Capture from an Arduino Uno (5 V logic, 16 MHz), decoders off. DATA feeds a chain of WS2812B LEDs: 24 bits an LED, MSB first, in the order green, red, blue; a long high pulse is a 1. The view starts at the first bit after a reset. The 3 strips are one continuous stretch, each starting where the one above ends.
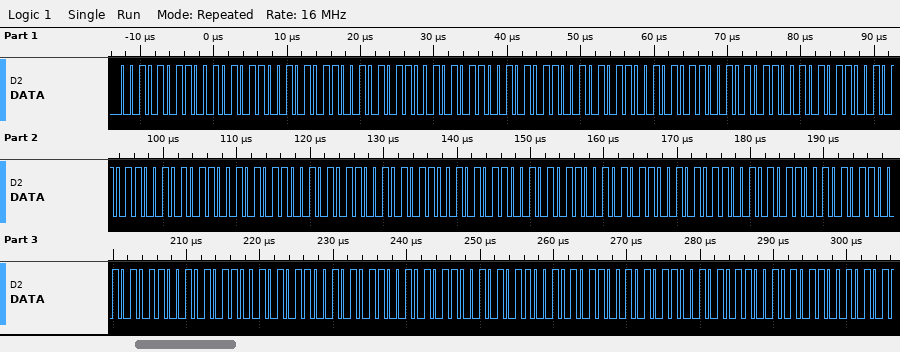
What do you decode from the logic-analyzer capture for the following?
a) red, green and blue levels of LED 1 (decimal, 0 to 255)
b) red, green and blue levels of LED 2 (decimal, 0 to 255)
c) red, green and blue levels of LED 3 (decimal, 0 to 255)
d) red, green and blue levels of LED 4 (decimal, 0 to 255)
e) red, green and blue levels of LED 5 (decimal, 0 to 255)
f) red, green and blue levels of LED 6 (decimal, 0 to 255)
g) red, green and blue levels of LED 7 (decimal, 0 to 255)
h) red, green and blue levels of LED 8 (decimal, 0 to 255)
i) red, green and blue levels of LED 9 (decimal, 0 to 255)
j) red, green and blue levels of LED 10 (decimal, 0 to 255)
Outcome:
43, 43, 43
43, 43, 43
43, 43, 43
43, 43, 43
43, 43, 43
43, 43, 43
43, 43, 43
43, 43, 43
43, 43, 43
43, 43, 43
